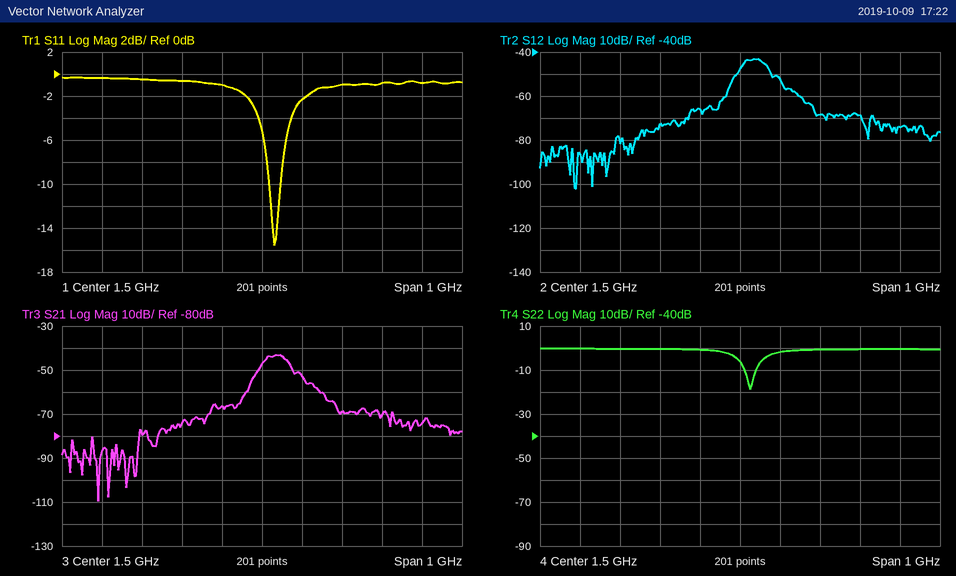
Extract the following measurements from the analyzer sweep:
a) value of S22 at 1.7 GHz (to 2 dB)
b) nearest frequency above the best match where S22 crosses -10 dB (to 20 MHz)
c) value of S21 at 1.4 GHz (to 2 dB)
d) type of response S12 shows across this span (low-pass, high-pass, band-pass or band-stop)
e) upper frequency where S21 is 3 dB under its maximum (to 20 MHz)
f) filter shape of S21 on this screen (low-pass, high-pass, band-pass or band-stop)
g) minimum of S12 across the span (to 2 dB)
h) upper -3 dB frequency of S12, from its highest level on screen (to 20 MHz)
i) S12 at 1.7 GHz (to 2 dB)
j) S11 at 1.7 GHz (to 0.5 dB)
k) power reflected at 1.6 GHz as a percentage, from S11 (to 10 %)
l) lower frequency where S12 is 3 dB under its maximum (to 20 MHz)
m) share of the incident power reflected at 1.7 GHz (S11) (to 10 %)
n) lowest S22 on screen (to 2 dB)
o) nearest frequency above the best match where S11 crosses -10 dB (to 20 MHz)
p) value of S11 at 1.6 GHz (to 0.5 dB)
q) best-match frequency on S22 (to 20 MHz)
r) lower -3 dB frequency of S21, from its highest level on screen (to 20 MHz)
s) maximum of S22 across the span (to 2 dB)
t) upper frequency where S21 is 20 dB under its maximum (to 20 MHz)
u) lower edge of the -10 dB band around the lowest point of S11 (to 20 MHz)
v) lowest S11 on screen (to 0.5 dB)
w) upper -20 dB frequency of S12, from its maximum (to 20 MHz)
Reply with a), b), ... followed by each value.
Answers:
a) 0 dB
b) 1.54 GHz
c) -66 dB
d) band-pass
e) 1.56 GHz
f) band-pass
g) -102 dB
h) 1.56 GHz
i) -68 dB
j) -1.0 dB
k) 60 %
l) 1.50 GHz
m) 80 %
n) -18 dB
o) 1.54 GHz
p) -2.5 dB
q) 1.52 GHz
r) 1.50 GHz
s) 0 dB
t) 1.66 GHz
u) 1.52 GHz
v) -15.5 dB
w) 1.66 GHz
